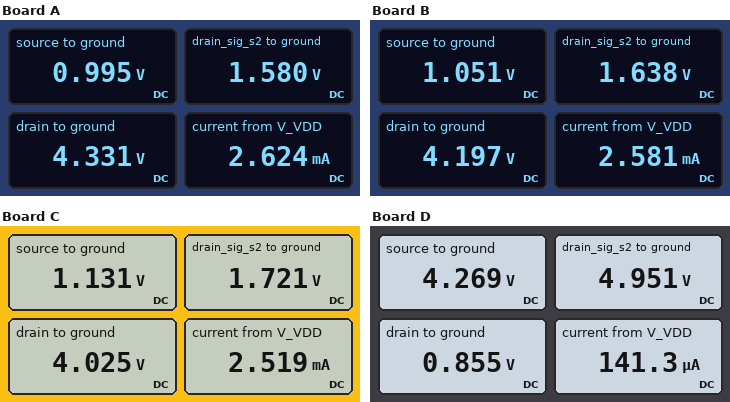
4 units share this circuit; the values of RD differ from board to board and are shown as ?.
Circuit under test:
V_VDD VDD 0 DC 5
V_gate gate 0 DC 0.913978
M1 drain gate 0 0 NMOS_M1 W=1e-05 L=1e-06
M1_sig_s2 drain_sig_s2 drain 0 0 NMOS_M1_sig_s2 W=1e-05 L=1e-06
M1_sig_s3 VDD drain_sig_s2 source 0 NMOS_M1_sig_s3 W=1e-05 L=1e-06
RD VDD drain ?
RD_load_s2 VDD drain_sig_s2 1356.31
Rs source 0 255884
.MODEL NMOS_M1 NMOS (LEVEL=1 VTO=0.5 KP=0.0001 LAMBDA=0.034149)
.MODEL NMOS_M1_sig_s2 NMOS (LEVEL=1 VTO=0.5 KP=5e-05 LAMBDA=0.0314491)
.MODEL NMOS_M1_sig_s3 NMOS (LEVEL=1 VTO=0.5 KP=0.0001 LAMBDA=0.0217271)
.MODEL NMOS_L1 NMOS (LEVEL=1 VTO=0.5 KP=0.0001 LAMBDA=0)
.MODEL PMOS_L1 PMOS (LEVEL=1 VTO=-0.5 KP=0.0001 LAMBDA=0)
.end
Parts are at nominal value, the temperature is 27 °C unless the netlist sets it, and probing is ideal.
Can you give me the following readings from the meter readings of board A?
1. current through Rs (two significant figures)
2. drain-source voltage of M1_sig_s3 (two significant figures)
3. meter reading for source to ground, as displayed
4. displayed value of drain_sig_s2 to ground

3.9 µA
4.0 V
0.995 V
1.580 V
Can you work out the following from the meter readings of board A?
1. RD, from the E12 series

6.8 kΩ
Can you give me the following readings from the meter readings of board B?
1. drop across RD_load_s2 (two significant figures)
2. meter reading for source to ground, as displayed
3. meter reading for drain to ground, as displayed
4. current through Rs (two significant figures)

3.4 V
1.051 V
4.197 V
4.1 µA
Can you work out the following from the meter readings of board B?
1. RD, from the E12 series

8.2 kΩ
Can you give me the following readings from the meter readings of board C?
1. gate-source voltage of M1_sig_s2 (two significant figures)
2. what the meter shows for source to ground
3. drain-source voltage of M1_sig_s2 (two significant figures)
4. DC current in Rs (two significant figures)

4.0 V
1.131 V
1.7 V
4.4 µA
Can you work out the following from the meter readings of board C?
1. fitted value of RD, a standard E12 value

10 kΩ
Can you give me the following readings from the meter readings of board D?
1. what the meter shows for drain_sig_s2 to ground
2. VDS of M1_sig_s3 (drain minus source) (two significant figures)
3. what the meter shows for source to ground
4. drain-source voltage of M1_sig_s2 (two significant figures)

4.951 V
730 mV
4.269 V
5.0 V
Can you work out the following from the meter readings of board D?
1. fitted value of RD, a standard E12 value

47 kΩ
